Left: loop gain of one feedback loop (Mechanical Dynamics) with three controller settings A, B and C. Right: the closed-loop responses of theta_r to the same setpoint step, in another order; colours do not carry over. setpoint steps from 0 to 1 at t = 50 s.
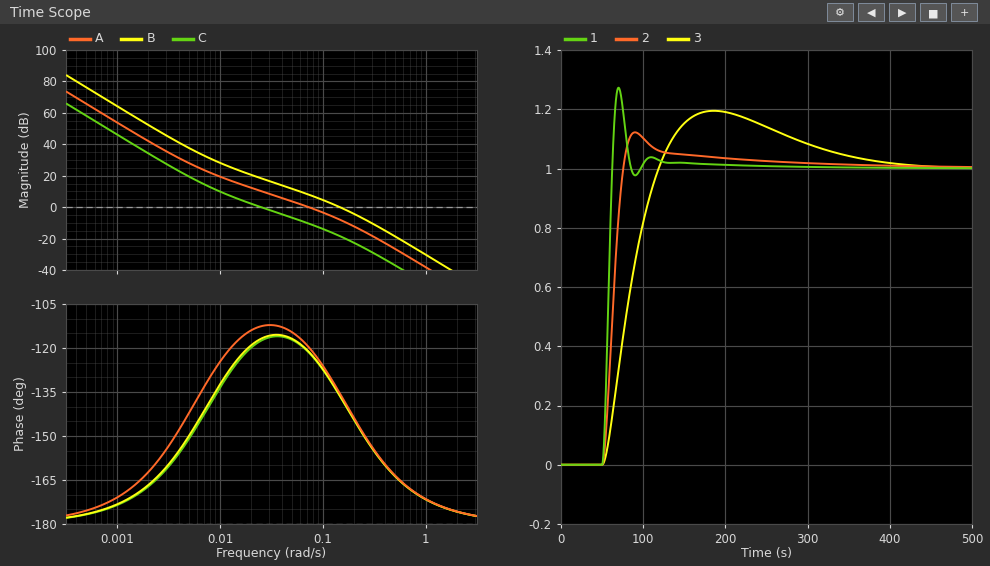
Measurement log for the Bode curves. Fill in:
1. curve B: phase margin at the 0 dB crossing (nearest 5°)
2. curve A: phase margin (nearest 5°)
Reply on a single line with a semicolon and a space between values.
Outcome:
45°; 60°
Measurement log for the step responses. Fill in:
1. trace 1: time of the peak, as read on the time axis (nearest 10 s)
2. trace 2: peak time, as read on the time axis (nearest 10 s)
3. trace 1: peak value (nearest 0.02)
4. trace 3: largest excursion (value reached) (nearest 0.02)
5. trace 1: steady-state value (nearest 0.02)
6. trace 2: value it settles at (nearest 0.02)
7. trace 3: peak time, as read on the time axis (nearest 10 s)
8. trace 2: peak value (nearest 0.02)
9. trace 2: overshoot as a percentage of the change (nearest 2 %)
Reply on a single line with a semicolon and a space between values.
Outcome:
70 s; 90 s; 1.28; 1.20; 1.00; 1.00; 190 s; 1.12; 12 %
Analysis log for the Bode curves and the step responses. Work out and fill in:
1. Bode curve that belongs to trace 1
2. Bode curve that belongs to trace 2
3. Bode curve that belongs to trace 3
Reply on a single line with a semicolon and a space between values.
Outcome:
B; A; C
